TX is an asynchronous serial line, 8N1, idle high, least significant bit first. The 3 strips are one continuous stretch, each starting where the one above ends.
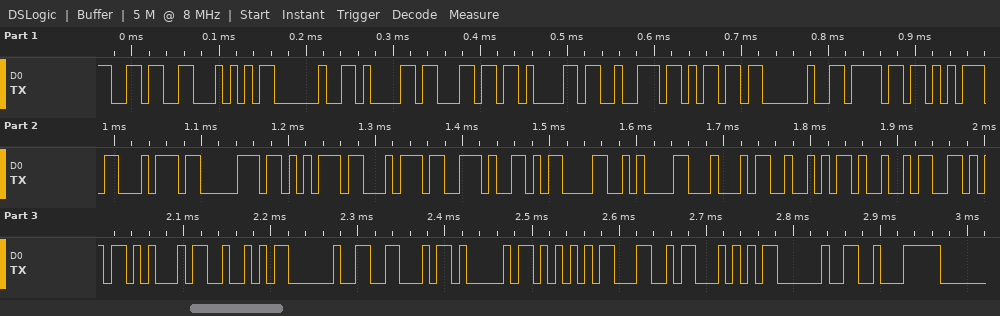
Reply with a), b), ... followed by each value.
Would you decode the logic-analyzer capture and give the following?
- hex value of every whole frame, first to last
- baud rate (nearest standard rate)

a) 36 54 20 61 6C 61 72 6D 20 6F 75 74 70 75 74 2E 0D 0A 44 52 49 56 45 52 20 46 41 55 4C 54 20 E2
b) 115200 baud
